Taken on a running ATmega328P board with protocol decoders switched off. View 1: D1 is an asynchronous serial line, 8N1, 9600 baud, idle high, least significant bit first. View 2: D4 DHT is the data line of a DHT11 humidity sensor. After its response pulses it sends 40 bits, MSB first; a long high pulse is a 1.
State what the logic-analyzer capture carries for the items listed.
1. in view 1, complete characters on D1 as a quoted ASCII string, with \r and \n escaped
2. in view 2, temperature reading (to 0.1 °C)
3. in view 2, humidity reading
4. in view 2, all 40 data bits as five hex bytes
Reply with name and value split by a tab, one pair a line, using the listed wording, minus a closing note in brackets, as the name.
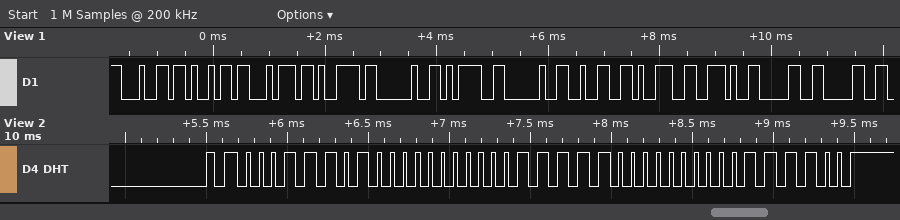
in view 1, complete characters on D1 as a quoted ASCII string, with \r and \n escaped	"dity = 29.00"
in view 2, temperature reading	31.0 °C
in view 2, humidity reading	29 %
in view 2, all 40 data bits as five hex bytes	1D 00 1F 00 3C
